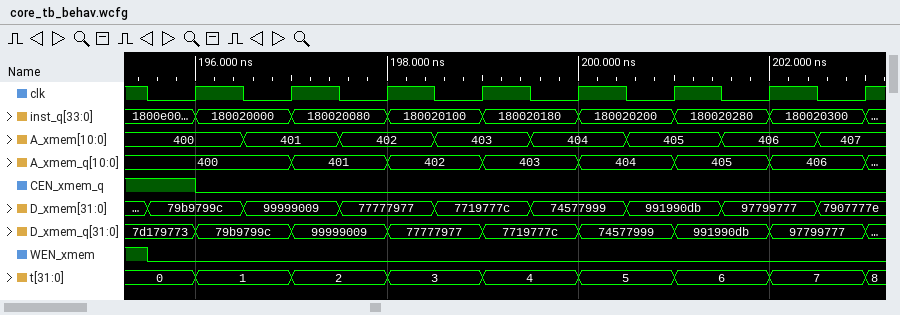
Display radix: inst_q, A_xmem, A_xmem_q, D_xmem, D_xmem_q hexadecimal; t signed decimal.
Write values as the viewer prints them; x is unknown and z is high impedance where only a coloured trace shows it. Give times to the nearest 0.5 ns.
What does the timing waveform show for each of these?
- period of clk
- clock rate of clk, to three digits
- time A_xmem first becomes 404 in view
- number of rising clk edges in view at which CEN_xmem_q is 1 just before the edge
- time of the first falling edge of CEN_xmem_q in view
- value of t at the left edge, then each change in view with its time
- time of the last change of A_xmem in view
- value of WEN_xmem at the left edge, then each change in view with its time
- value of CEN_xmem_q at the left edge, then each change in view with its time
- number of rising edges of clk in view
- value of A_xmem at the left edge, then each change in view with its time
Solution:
1 ns
1.00 GHz
199.5 ns
1
196 ns
0, 1 at 196 ns, 2 at 197 ns, 3 at 198 ns, 4 at 199 ns, 5 at 200 ns, 6 at 201 ns, 7 at 202 ns, 8 at 203 ns
202.5 ns
1, 0 at 195.5 ns
1, 0 at 196 ns
8
400, 401 at 196.5 ns, 402 at 197.5 ns, 403 at 198.5 ns, 404 at 199.5 ns, 405 at 200.5 ns, 406 at 201.5 ns, 407 at 202.5 ns
